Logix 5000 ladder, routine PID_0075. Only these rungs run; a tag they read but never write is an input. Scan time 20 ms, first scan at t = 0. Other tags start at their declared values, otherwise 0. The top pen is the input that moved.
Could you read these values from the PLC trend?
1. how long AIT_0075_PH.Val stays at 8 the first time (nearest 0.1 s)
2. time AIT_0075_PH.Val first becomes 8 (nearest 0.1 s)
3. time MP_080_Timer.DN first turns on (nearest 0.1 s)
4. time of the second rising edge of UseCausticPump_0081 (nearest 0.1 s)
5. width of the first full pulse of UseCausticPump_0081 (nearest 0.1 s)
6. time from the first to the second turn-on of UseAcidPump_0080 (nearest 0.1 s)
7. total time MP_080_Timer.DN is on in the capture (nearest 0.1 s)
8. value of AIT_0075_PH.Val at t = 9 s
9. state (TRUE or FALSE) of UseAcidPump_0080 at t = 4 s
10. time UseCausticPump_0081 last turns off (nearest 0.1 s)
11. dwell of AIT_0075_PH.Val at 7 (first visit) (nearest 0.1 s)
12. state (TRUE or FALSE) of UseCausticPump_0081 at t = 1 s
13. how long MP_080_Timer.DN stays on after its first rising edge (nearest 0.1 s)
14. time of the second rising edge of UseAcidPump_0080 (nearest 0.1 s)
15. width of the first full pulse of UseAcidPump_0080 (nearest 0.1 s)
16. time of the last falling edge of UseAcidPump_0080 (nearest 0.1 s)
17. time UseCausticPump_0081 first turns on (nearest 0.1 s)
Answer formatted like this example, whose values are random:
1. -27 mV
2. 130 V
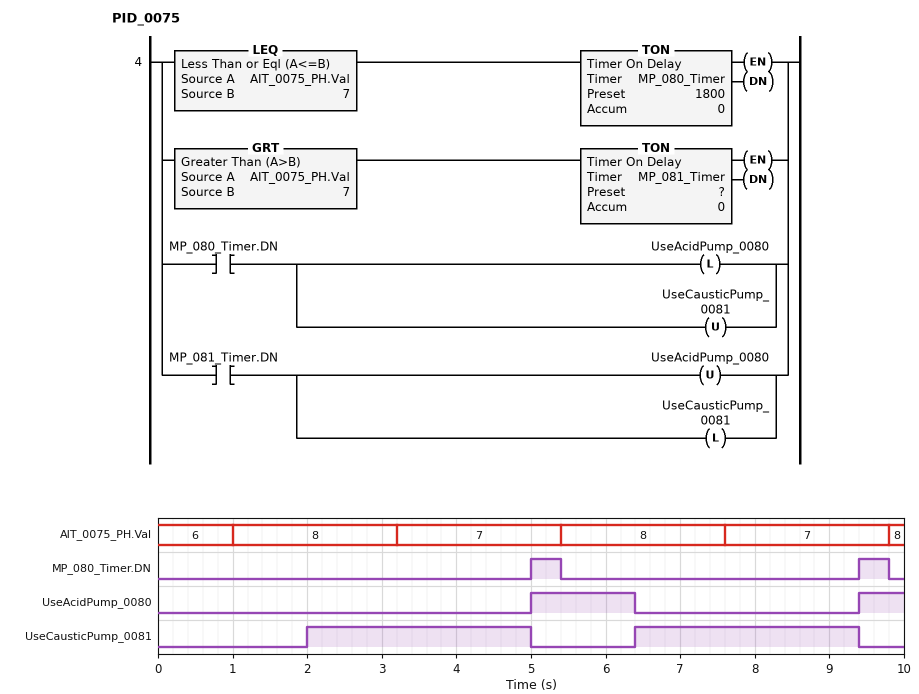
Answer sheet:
1. 2.2 s
2. 1.0 s
3. 5.0 s
4. 6.4 s
5. 3.0 s
6. 4.4 s
7. 0.8 s
8. 7
9. FALSE
10. 9.4 s
11. 2.2 s
12. FALSE
13. 0.4 s
14. 9.4 s
15. 1.4 s
16. 6.4 s
17. 2.0 s
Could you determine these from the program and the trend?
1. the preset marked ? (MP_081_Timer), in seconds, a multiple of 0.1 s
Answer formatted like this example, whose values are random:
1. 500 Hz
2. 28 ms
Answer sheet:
1. 1.0 s
